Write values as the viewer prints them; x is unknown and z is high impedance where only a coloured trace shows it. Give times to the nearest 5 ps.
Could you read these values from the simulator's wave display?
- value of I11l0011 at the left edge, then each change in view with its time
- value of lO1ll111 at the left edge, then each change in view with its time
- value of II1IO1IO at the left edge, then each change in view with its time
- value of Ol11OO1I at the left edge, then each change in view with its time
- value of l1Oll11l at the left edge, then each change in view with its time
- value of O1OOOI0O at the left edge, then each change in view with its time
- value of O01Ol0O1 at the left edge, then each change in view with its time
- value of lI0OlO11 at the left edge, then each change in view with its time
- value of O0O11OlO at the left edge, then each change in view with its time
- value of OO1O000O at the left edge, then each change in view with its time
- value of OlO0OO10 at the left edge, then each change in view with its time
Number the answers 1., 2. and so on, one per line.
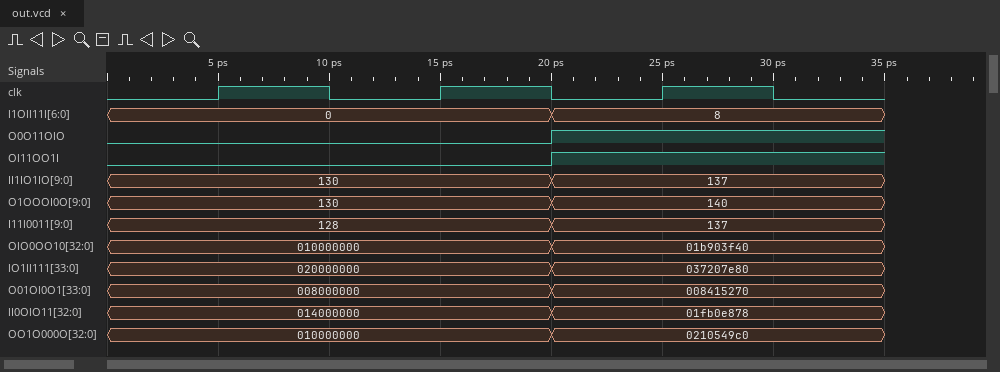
1. 128, 137 at 20 ps
2. 020000000, 037207e80 at 20 ps
3. 130, 137 at 20 ps
4. 0, 1 at 20 ps
5. 0, 8 at 20 ps
6. 130, 140 at 20 ps
7. 008000000, 008415270 at 20 ps
8. 014000000, 01fb0e878 at 20 ps
9. 0, 1 at 20 ps
10. 010000000, 0210549c0 at 20 ps
11. 010000000, 01b903f40 at 20 ps
